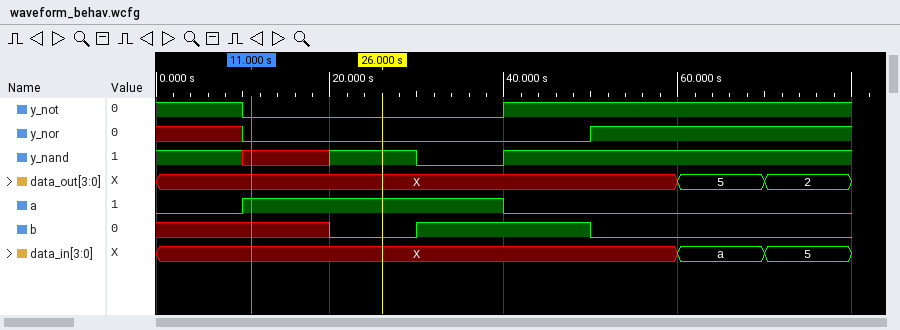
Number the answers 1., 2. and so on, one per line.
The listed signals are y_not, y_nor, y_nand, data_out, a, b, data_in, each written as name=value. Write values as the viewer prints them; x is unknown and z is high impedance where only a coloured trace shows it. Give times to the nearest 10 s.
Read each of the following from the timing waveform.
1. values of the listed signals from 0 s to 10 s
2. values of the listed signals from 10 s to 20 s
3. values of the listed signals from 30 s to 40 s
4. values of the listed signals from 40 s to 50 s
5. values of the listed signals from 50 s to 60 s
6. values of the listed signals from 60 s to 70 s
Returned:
1. y_not=1, y_nor=x, y_nand=1, data_out=X, a=0, b=x, data_in=X
2. y_not=0, y_nor=0, y_nand=x, data_out=X, a=1, b=x, data_in=X
3. y_not=0, y_nor=0, y_nand=0, data_out=X, a=1, b=1, data_in=X
4. y_not=1, y_nor=0, y_nand=1, data_out=X, a=0, b=1, data_in=X
5. y_not=1, y_nor=1, y_nand=1, data_out=X, a=0, b=0, data_in=X
6. y_not=1, y_nor=1, y_nand=1, data_out=5, a=0, b=0, data_in=a
